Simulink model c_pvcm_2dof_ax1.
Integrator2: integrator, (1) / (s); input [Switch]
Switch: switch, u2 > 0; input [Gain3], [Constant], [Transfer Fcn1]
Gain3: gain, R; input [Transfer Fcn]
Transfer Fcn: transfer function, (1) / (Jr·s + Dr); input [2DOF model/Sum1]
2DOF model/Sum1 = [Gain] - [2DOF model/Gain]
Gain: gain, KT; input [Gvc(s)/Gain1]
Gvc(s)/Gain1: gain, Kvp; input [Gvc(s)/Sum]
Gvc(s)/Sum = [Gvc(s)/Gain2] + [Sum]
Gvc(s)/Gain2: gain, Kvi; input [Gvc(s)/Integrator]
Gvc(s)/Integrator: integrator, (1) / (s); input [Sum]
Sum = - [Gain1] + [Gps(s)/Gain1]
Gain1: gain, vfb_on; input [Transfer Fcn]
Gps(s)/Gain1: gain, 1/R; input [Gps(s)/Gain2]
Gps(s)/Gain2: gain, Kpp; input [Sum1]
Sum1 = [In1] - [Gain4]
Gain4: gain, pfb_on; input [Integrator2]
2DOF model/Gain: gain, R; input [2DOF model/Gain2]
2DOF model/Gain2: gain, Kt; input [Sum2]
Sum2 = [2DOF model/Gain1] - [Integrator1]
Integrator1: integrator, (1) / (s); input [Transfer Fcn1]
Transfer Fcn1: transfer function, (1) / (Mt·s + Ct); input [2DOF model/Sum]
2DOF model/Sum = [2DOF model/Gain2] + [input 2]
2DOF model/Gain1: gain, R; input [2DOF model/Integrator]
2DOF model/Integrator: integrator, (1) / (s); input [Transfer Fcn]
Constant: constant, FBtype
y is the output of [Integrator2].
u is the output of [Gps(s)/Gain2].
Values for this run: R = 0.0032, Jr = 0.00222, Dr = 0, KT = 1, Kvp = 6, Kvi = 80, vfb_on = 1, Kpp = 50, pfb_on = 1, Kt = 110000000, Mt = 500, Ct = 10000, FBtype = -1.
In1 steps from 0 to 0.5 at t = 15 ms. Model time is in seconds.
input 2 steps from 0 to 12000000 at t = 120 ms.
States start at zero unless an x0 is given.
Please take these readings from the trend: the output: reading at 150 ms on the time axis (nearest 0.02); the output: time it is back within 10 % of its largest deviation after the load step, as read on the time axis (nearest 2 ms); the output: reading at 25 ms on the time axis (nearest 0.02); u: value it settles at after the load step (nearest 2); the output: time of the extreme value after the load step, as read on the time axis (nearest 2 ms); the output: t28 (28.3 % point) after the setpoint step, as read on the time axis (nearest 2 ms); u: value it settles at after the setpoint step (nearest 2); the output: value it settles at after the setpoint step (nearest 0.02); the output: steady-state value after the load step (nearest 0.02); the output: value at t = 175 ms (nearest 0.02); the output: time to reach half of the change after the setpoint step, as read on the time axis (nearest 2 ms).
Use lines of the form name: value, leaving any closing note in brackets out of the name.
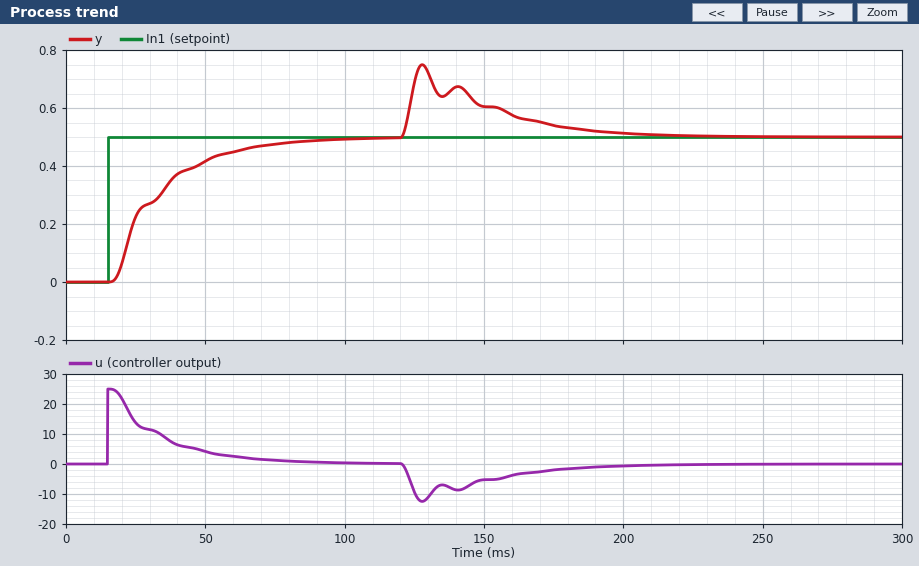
the output: reading at 150 ms on the time axis: 0.60
the output: time it is back within 10 % of its largest deviation after the load step, as read on the time axis: 186 ms
the output: reading at 25 ms on the time axis: 0.22
u: value it settles at after the load step: 0
the output: time of the extreme value after the load step, as read on the time axis: 128 ms
the output: t28 (28.3 % point) after the setpoint step, as read on the time axis: 22 ms
u: value it settles at after the setpoint step: 0
the output: value it settles at after the setpoint step: 0.50
the output: steady-state value after the load step: 0.50
the output: value at t = 175 ms: 0.54
the output: time to reach half of the change after the setpoint step, as read on the time axis: 26 ms
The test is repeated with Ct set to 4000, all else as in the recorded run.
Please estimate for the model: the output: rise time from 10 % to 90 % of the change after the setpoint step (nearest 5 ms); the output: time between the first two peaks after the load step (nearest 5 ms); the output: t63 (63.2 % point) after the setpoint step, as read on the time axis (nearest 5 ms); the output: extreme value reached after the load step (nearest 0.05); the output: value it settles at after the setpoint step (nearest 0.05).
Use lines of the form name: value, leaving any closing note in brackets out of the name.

the output: rise time from 10 % to 90 % of the change after the setpoint step: 40 ms
the output: time between the first two peaks after the load step: 15 ms
the output: t63 (63.2 % point) after the setpoint step, as read on the time axis: 35 ms
the output: extreme value reached after the load step: 0.75
the output: value it settles at after the setpoint step: 0.50
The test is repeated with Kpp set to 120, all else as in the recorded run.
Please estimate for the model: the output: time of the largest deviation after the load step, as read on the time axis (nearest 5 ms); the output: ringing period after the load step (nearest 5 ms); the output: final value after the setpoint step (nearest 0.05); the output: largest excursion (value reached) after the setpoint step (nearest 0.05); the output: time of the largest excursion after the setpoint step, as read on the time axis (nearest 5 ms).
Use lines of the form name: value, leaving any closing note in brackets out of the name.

the output: time of the largest deviation after the load step, as read on the time axis: 125 ms
the output: ringing period after the load step: 15 ms
the output: final value after the setpoint step: 0.50
the output: largest excursion (value reached) after the setpoint step: 0.55
the output: time of the largest excursion after the setpoint step, as read on the time axis: 40 ms
